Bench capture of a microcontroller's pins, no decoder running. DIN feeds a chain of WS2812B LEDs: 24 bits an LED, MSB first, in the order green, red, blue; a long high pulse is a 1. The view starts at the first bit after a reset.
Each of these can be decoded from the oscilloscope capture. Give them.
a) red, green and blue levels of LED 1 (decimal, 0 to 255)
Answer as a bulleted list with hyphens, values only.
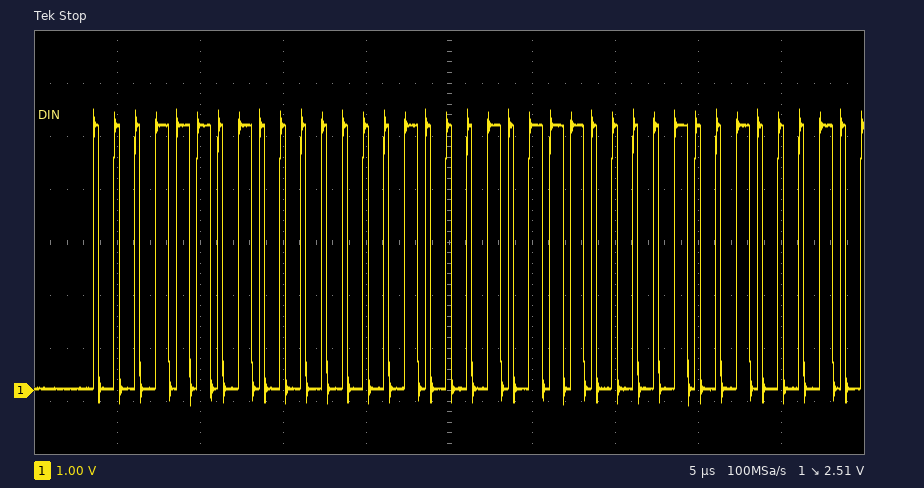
- 1, 29, 23
